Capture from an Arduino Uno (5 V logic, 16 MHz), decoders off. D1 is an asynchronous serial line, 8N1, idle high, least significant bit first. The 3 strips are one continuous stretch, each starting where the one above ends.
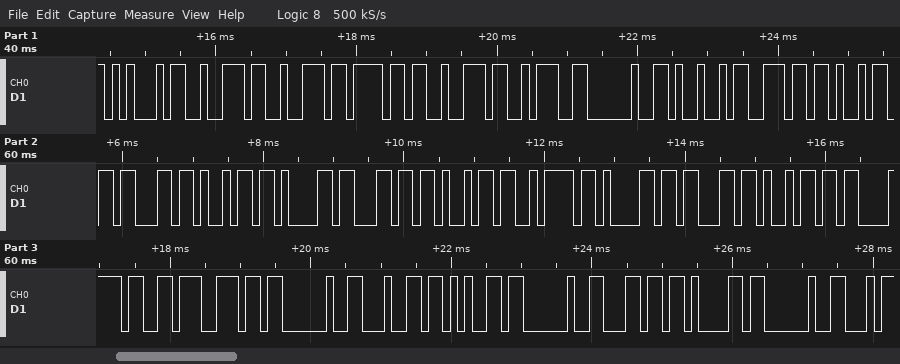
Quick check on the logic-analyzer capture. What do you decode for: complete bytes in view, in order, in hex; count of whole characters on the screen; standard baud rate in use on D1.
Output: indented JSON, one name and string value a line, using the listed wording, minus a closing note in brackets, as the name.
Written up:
{
  "complete bytes in view, in order, in hex": "45 72 72 6F 72 3A 20 49 6E 69 63 69 61 6C 69 7A 61 63 69 C3 B3 6E 20 64 65 20 6C 61 20",
  "count of whole characters on the screen": "29",
  "standard baud rate in use on D1": "9600 baud"
}
